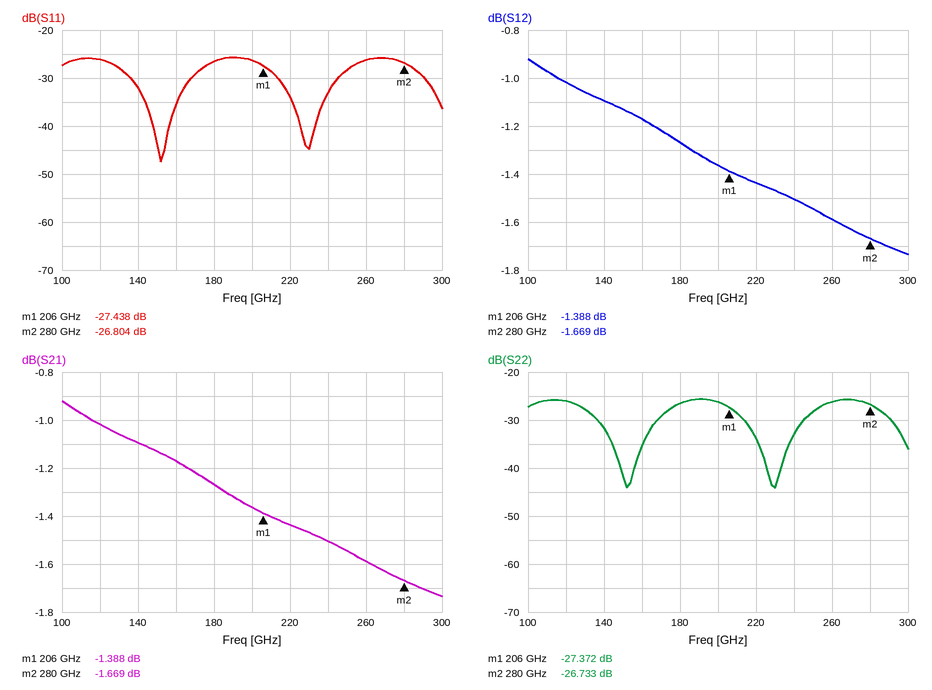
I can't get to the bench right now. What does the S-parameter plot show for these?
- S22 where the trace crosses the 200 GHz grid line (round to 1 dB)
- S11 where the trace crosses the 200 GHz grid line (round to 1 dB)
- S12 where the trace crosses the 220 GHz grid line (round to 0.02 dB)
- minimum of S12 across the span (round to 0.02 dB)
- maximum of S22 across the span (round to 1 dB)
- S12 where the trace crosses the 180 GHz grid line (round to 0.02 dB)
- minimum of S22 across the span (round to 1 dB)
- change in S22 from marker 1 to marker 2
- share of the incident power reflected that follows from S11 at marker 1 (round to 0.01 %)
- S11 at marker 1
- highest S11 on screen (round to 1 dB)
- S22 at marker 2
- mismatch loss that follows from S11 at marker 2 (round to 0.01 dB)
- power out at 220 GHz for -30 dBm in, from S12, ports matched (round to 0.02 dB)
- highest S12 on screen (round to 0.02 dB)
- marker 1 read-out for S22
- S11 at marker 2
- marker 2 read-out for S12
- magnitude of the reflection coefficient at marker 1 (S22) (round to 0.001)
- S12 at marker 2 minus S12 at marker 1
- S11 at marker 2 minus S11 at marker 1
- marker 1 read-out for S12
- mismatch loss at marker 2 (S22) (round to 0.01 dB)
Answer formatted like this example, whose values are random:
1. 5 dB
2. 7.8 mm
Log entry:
1. -26 dB
2. -26 dB
3. -1.44 dB
4. -1.74 dB
5. -26 dB
6. -1.26 dB
7. -44 dB
8. 0.639 dB
9. 0.18 %
10. -27.438 dB
11. -26 dB
12. -26.733 dB
13. 0.01 dB
14. -31.44 dBm
15. -0.92 dB
16. -27.372 dB
17. -26.804 dB
18. -1.669 dB
19. 0.043
20. -0.281 dB
21. 0.634 dB
22. -1.388 dB
23. 0.01 dB
